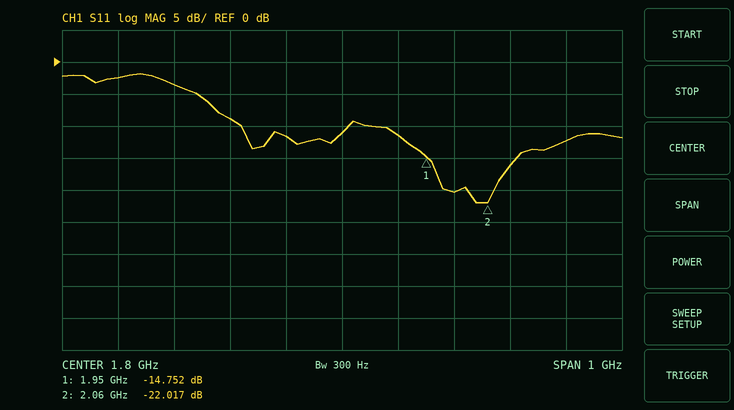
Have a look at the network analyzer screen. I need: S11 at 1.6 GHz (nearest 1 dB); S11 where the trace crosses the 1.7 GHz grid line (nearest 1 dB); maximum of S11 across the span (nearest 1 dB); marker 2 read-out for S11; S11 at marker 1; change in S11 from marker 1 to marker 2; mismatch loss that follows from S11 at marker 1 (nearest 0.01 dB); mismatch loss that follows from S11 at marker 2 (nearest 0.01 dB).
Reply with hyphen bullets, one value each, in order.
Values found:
- -9 dB
- -12 dB
- -2 dB
- -22.017 dB
- -14.752 dB
- -7.265 dB
- 0.15 dB
- 0.03 dB
